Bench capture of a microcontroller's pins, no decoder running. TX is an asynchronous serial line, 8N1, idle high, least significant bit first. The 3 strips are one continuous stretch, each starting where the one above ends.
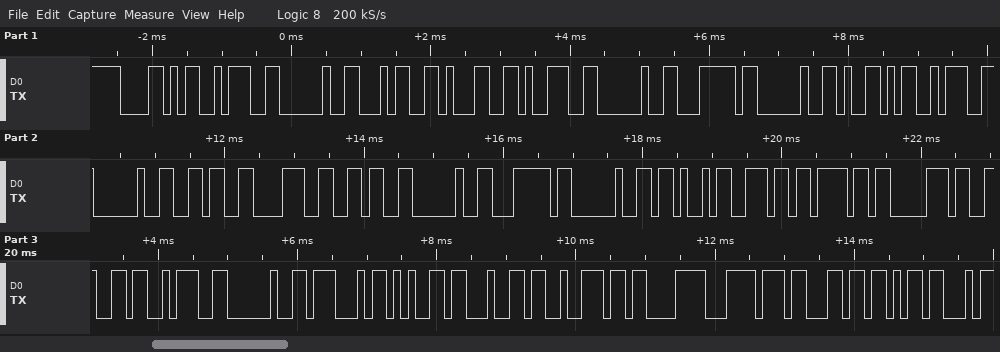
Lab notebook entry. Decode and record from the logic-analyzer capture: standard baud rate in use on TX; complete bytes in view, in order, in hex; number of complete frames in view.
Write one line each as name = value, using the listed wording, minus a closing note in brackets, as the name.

standard baud rate in use on TX = 9600 baud
complete bytes in view, in order, in hex = 58 3A 20 34 31 39 20 7C 20 59 3A 20 36 38 36 20 7C 20 4B 6E 6F 70 66 3A 20 47 65 64 72 C3 BC 63 6B
number of complete frames in view = 33
